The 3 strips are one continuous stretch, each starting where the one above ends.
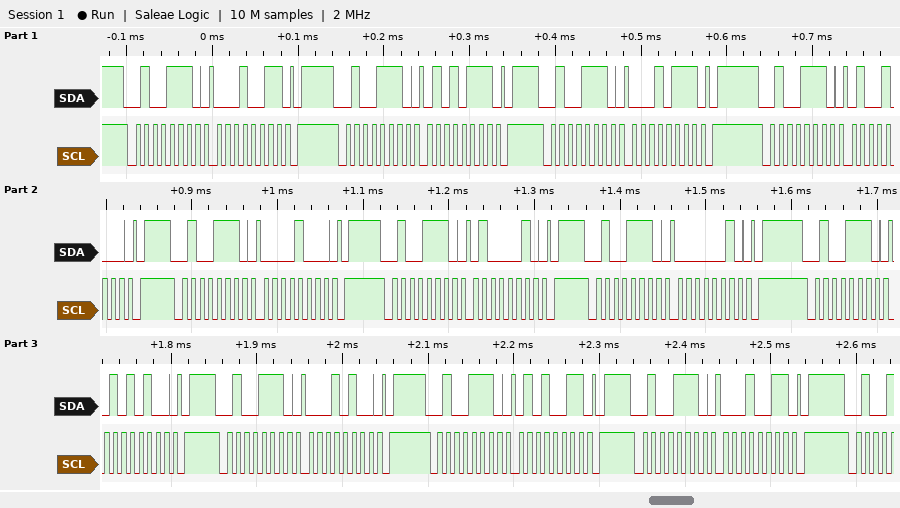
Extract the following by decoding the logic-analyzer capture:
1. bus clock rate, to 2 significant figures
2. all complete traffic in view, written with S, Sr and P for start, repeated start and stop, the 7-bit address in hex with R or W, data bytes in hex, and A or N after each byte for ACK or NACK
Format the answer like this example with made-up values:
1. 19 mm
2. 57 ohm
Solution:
1. 100 kHz
2. S 27W A 13 A P S 27W A 57 A P S 27W A 17 A P S 27W A 48 A P S 27W A 08 A P S 27W A 42 A P S 27W A 02 A P S 27W A 54 A P S 27W A 14 A P S 27W A 53 A P S 27W A 13 A P
